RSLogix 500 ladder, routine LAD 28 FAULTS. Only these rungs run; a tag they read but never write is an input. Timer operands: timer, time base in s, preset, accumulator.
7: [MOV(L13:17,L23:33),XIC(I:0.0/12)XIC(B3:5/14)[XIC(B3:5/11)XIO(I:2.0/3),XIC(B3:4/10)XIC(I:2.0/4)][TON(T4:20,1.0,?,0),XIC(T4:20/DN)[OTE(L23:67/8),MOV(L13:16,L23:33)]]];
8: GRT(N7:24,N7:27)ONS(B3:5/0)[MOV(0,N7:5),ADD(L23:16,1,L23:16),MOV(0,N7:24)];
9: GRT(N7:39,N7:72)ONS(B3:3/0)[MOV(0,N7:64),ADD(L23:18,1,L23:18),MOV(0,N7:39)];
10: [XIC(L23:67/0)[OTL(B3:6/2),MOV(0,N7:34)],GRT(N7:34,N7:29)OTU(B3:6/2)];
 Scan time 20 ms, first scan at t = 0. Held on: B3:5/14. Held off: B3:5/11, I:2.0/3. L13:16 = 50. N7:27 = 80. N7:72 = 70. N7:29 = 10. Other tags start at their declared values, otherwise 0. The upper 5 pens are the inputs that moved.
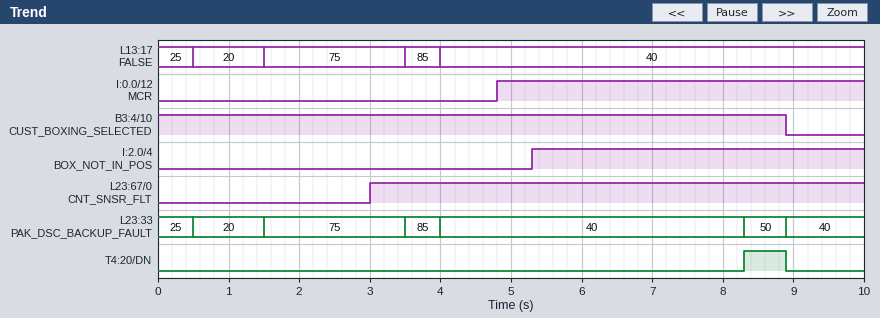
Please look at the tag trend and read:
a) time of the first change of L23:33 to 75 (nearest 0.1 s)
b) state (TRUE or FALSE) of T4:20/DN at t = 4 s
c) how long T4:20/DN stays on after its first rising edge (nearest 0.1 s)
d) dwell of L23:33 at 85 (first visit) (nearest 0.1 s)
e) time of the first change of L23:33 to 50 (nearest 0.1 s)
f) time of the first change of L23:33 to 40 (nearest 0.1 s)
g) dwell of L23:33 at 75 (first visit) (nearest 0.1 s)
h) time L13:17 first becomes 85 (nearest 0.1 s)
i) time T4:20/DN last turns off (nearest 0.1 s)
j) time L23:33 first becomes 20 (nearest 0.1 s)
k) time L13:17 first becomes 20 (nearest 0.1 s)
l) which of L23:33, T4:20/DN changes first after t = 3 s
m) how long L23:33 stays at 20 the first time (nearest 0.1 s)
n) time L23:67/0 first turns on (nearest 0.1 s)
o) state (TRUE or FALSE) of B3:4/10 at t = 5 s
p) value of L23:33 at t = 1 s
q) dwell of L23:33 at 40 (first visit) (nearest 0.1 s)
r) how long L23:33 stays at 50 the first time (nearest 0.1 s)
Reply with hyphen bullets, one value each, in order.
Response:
- 1.5 s
- FALSE
- 0.6 s
- 0.5 s
- 8.3 s
- 4.0 s
- 2.0 s
- 3.5 s
- 8.9 s
- 0.5 s
- 0.5 s
- L23:33
- 1.0 s
- 3.0 s
- TRUE
- 20
- 4.3 s
- 0.6 s
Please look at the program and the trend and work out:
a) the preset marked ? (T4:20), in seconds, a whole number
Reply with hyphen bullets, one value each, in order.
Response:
- 3 s
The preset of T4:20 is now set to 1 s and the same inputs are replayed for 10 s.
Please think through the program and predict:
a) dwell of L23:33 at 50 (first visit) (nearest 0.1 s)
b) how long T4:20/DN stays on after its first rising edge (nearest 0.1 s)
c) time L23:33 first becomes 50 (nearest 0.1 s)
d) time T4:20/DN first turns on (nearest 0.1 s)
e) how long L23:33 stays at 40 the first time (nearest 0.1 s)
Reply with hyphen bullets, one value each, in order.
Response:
- 2.6 s
- 2.6 s
- 6.3 s
- 6.3 s
- 2.3 s
